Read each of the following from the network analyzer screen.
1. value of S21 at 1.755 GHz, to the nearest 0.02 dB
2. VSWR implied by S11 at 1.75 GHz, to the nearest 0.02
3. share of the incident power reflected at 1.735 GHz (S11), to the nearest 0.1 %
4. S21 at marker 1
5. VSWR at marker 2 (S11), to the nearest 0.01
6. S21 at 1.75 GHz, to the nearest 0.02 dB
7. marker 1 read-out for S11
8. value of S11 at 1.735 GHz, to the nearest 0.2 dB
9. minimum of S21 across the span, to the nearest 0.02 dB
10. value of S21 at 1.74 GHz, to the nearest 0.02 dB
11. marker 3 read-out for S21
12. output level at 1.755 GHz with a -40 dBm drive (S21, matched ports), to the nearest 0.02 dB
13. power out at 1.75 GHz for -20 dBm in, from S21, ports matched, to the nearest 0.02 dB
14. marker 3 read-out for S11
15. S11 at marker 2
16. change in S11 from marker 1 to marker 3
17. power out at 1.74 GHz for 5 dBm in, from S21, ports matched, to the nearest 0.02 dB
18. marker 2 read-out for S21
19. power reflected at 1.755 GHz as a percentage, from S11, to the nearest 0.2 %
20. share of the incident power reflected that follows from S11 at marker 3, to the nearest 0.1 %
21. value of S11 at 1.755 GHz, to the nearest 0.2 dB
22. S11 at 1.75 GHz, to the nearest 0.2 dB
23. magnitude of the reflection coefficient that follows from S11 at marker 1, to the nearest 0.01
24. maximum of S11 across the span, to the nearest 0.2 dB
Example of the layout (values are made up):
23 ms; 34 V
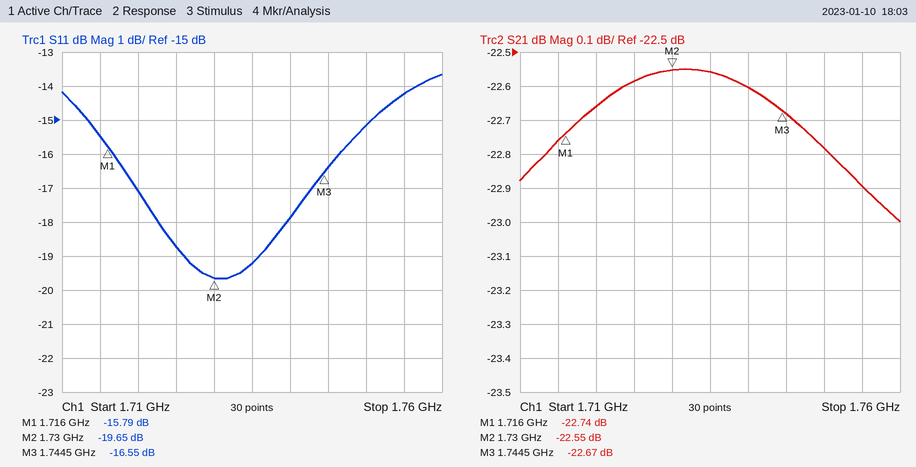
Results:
-22.90 dB; 1.42; 1.2 %; -22.74 dB; 1.23; -22.78 dB; -15.79 dB; -19.2 dB; -23.00 dB; -22.60 dB; -22.67 dB; -62.90 dBm; -42.78 dBm; -16.55 dB; -19.65 dB; -0.76 dB; -17.60 dBm; -22.55 dB; 3.8 %; 2.2 %; -14.2 dB; -15.2 dB; 0.16; -13.6 dB
